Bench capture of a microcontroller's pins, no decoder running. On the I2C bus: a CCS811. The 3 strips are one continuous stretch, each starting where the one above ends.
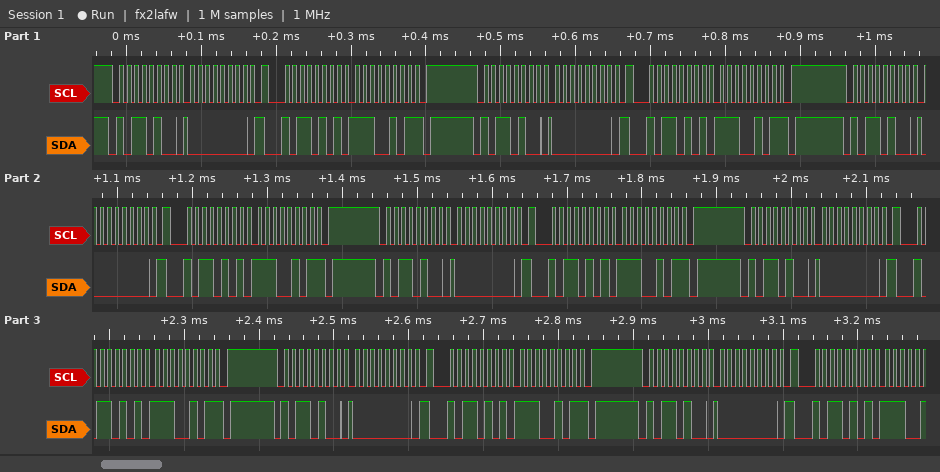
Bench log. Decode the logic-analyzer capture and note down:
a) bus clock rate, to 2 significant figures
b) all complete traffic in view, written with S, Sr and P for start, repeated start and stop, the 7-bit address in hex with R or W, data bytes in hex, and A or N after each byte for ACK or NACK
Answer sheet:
100 kHz
S 5AW A 00 A Sr 5AR A E5 N P S 5AW A 00 A Sr 5AR A E5 N P S 5AW A 00 A Sr 5AR A E5 N P S 5AW A 00 A Sr 5AR A E5 N P S 5AW A 00 A Sr 5AR A E5 N P S 5AW A 00 A Sr 5AR A E5 N P S 5AW A 00 A Sr 5AR A
